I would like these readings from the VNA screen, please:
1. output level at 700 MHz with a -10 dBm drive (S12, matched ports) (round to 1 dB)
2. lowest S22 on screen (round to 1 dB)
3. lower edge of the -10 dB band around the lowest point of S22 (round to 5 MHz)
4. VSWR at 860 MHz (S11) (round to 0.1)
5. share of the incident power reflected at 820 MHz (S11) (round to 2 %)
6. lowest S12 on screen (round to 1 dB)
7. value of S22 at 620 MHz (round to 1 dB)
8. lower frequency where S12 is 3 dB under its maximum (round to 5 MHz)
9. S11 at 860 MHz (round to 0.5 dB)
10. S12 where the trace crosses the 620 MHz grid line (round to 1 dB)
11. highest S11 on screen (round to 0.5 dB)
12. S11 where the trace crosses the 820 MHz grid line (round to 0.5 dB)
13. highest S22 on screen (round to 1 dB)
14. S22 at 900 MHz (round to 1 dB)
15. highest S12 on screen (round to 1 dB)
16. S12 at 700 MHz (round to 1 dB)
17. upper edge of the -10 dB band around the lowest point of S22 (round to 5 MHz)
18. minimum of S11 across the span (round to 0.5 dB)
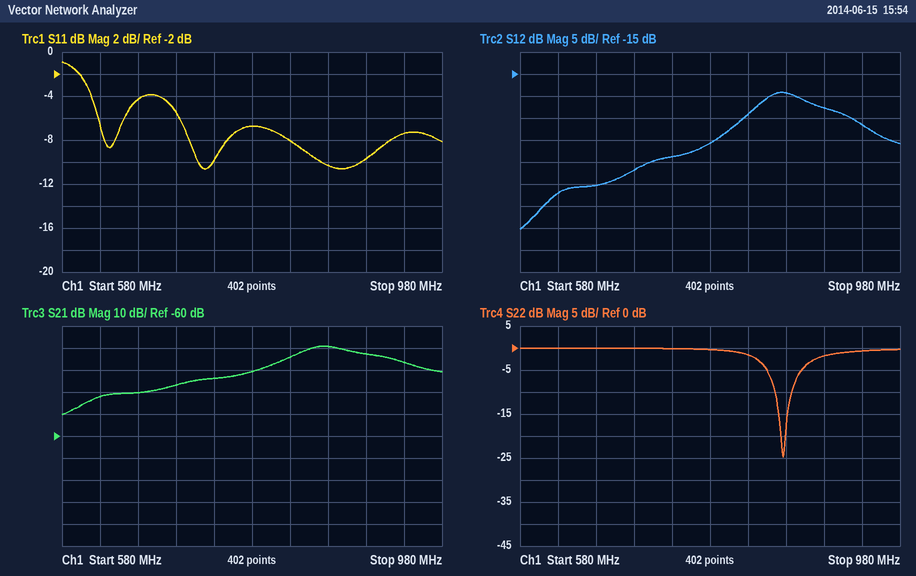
-47 dBm
-25 dB
850 MHz
1.9
16 %
-50 dB
0 dB
830 MHz
-10.5 dB
-42 dB
-1.0 dB
-8.0 dB
0 dB
-2 dB
-19 dB
-37 dB
865 MHz
-10.5 dB
